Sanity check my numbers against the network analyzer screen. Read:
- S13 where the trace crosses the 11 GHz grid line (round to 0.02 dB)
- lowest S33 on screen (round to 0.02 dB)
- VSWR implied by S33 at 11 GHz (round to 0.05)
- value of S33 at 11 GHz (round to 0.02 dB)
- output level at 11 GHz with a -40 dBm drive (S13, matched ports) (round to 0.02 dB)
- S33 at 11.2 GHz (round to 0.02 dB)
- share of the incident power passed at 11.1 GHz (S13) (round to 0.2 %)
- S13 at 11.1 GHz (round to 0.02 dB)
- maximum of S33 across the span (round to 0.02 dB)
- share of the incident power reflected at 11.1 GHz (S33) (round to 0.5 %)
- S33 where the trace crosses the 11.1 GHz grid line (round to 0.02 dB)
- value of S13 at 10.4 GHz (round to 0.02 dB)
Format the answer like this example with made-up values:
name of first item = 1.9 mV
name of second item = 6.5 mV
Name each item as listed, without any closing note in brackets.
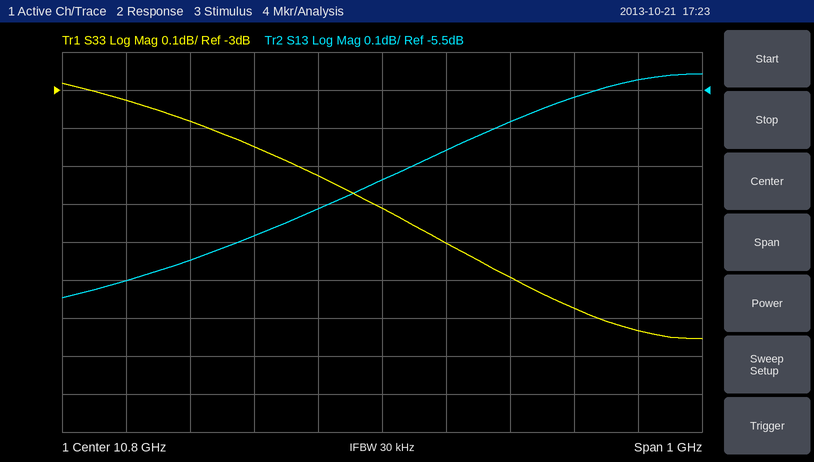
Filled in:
S13 where the trace crosses the 11 GHz grid line = -5.58 dB
lowest S33 on screen = -3.66 dB
VSWR implied by S33 at 11 GHz = 5.05
value of S33 at 11 GHz = -3.50 dB
output level at 11 GHz with a -40 dBm drive (S13, matched ports) = -45.58 dBm
S33 at 11.2 GHz = -3.64 dB
share of the incident power passed at 11.1 GHz (S13) = 28.0 %
S13 at 11.1 GHz = -5.52 dB
maximum of S33 across the span = -2.98 dB
share of the incident power reflected at 11.1 GHz (S33) = 44.0 %
S33 where the trace crosses the 11.1 GHz grid line = -3.58 dB
value of S13 at 10.4 GHz = -6.00 dB
